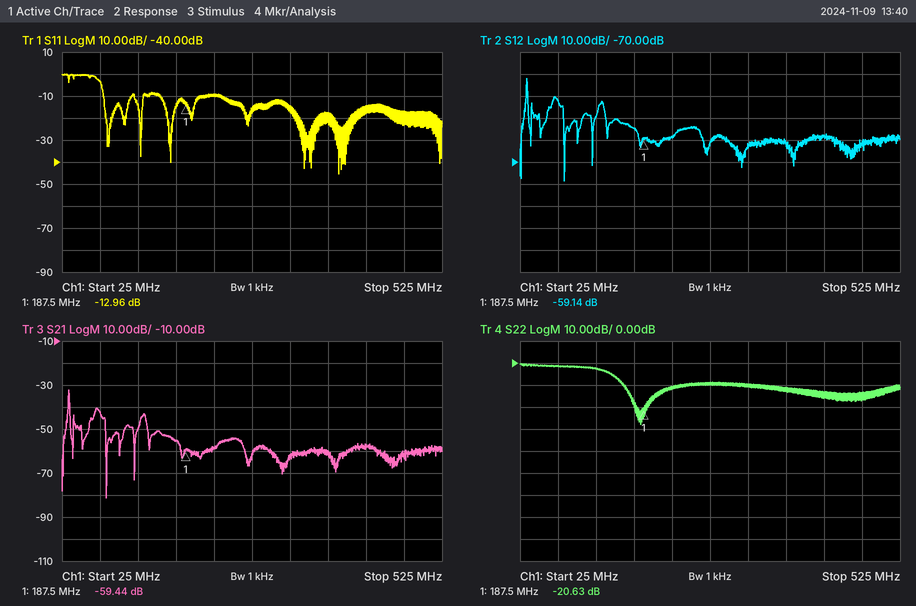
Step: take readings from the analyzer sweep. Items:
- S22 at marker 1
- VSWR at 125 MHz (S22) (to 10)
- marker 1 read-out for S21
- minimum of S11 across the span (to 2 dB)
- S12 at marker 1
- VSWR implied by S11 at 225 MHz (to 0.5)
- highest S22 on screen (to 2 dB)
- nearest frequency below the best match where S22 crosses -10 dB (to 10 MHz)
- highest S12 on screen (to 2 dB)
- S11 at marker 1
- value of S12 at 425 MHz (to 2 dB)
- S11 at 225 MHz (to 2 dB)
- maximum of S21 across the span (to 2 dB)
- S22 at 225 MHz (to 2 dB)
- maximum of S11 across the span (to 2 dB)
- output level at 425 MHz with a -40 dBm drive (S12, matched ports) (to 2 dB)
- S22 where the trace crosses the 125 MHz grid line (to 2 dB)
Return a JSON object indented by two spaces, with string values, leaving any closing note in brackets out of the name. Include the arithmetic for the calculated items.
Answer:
{
  "S22 at marker 1": "-20.63 dB",
  "VSWR at 125 MHz (S22)": "|Γ| = 10^(-2/20) = 0.7943; VSWR = (1 + 0.7943)/(1 − 0.7943) ≈ 8.72, so 10 to the nearest 10",
  "marker 1 read-out for S21": "-59.44 dB",
  "minimum of S11 across the span": "-46 dB",
  "S12 at marker 1": "-59.14 dB",
  "VSWR implied by S11 at 225 MHz": "|Γ| = 10^(-10/20) = 0.3162; VSWR = (1 + 0.3162)/(1 − 0.3162) ≈ 1.92, so 2.0 to the nearest 0.5",
  "highest S22 on screen": "0 dB",
  "nearest frequency below the best match where S22 crosses -10 dB": "160 MHz",
  "highest S12 on screen": "-32 dB",
  "S11 at marker 1": "-12.96 dB",
  "value of S12 at 425 MHz": "-58 dB",
  "S11 at 225 MHz": "-10 dB",
  "maximum of S21 across the span": "-32 dB",
  "S22 at 225 MHz": "-12 dB",
  "maximum of S11 across the span": "0 dB",
  "output level at 425 MHz with a -40 dBm drive (S12, matched ports)": "-40 dBm + (-58 dB) = -98 dBm",
  "S22 where the trace crosses the 125 MHz grid line": "-2 dB"
}
